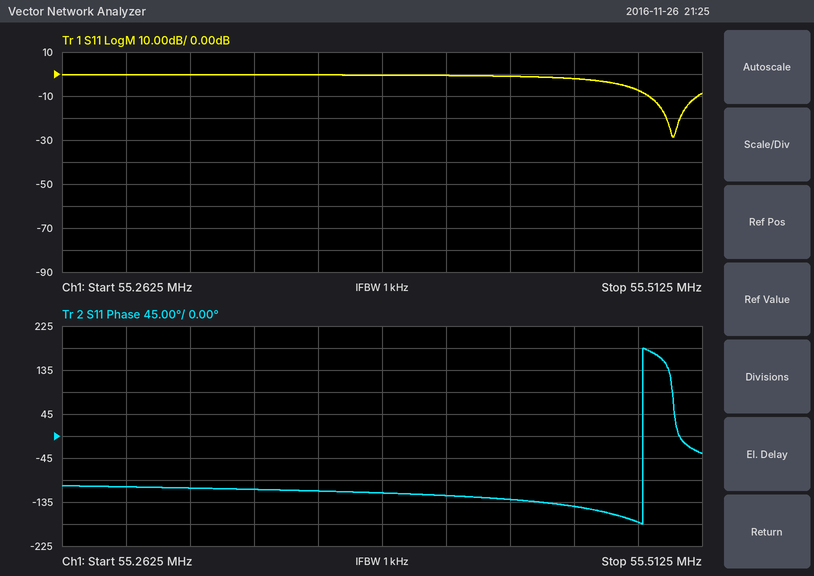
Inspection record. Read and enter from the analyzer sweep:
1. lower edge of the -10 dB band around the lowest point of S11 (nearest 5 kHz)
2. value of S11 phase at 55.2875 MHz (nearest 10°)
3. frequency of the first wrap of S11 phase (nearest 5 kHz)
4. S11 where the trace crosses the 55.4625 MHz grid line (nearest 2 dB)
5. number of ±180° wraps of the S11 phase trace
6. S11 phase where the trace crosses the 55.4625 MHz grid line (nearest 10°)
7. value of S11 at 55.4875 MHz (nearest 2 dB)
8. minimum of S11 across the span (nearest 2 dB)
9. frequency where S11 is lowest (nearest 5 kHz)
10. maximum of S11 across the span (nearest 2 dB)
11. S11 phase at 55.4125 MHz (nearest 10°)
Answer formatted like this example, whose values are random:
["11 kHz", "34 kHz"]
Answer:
["55.490 MHz", "-100°", "55.490 MHz", "-2 dB", "1", "-140°", "-8 dB", "-28 dB", "55.500 MHz", "0 dB", "-120°"]
